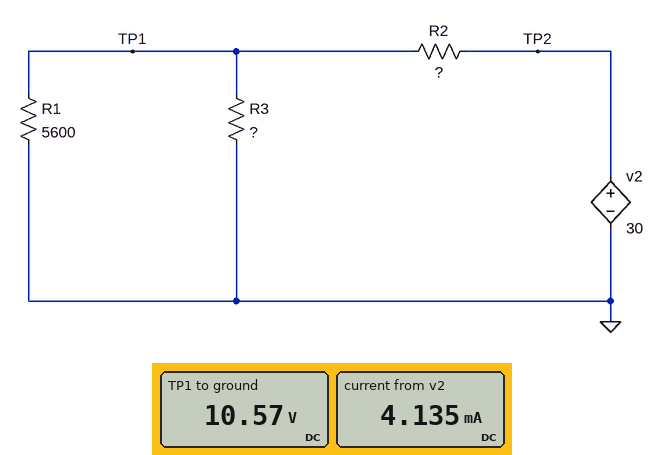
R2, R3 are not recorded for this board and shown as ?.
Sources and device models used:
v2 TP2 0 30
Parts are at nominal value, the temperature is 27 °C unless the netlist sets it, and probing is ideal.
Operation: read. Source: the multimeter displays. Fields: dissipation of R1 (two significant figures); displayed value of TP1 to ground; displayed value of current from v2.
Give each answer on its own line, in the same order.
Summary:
20 mW
10.57 V
4.135 mA
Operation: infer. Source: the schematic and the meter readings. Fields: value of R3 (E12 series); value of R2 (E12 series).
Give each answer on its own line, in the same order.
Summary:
4.7 kΩ
4.7 kΩ
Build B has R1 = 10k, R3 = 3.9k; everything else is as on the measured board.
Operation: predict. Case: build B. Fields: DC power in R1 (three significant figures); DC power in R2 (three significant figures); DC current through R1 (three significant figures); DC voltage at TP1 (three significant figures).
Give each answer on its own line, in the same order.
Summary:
12.6 mW
75.1 mW
1.12 mA
11.2 V
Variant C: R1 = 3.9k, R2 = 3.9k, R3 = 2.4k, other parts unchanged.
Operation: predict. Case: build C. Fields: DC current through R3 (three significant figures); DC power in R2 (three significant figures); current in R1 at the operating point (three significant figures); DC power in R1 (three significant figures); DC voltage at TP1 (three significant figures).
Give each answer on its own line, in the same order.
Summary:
3.45 mA
121 mW
2.12 mA
17.6 mW
8.28 V
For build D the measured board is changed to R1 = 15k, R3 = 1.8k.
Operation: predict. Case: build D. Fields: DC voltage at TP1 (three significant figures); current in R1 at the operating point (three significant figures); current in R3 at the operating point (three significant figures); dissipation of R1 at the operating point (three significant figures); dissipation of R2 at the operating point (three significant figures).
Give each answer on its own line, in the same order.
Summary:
7.64 V
510 µA
4.25 mA
3.90 mW
106 mW
